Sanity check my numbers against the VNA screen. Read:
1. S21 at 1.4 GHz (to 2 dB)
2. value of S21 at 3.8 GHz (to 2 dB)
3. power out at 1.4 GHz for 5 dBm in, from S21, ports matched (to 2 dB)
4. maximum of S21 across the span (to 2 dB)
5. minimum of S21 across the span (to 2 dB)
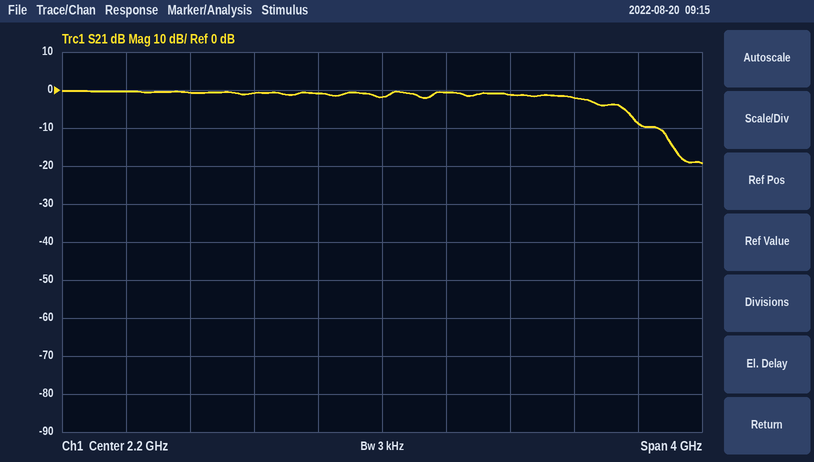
0 dB
-8 dB
4 dBm
0 dB
-20 dB
